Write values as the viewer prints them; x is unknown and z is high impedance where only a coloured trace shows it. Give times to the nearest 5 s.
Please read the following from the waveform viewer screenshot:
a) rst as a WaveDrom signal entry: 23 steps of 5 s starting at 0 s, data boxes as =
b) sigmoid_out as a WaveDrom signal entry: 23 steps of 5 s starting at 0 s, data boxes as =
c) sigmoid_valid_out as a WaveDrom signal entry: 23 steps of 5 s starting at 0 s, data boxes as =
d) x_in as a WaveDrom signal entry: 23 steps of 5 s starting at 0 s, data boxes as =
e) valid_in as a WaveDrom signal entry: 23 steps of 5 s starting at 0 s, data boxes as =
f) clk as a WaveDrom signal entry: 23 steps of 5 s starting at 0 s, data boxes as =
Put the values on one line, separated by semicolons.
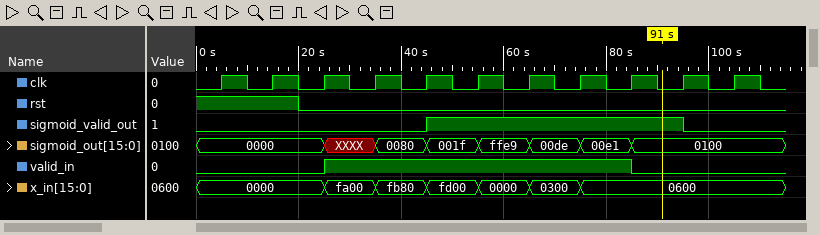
{name: 'rst', wave: '1...0..................'}; {name: 'sigmoid_out', wave: '=....x.=.=.=.=.=.=.....', data: '0000 0080 001f ffe9 00de 00e1 0100'}; {name: 'sigmoid_valid_out', wave: '0........1.........0...'}; {name: 'x_in', wave: '=....=.=.=.=.=.=.......', data: '0000 fa00 fb80 fd00 0000 0300 0600'}; {name: 'valid_in', wave: '0....1...........0.....'}; {name: 'clk', wave: '01010101010101010101010'}
